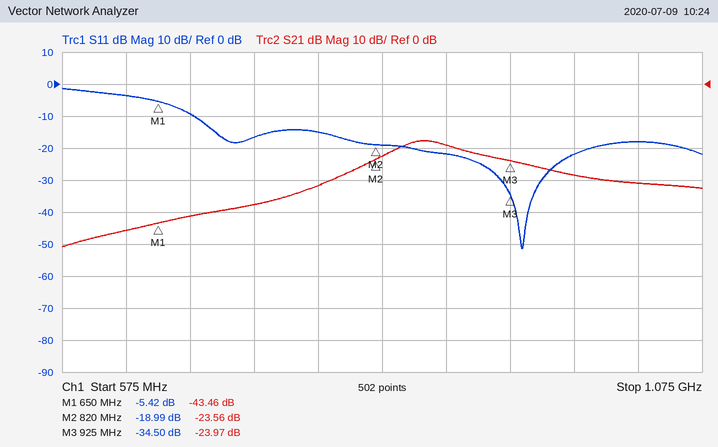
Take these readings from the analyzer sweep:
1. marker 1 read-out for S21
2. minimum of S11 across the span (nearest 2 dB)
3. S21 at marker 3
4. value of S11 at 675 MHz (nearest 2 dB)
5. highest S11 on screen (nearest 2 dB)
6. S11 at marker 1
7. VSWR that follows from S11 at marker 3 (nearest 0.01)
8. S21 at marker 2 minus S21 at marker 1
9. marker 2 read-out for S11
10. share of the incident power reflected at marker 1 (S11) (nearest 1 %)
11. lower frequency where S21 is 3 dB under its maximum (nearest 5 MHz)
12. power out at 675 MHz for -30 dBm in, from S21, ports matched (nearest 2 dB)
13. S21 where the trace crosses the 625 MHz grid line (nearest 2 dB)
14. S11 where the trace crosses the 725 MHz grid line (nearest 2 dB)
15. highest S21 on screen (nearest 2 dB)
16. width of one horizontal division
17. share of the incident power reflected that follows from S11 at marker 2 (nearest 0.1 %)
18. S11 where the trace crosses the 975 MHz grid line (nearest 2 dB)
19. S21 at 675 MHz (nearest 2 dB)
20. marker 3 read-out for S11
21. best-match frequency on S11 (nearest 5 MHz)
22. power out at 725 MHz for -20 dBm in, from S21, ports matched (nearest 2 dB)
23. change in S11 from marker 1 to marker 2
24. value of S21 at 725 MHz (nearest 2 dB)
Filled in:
-43.46 dB
-52 dB
-23.97 dB
-10 dB
-2 dB
-5.42 dB
1.04
19.90 dB
-18.99 dB
29 %
835 MHz
-72 dBm
-46 dB
-16 dB
-18 dB
50 MHz
1.3 %
-22 dB
-42 dB
-34.50 dB
935 MHz
-58 dBm
-13.57 dB
-38 dB
